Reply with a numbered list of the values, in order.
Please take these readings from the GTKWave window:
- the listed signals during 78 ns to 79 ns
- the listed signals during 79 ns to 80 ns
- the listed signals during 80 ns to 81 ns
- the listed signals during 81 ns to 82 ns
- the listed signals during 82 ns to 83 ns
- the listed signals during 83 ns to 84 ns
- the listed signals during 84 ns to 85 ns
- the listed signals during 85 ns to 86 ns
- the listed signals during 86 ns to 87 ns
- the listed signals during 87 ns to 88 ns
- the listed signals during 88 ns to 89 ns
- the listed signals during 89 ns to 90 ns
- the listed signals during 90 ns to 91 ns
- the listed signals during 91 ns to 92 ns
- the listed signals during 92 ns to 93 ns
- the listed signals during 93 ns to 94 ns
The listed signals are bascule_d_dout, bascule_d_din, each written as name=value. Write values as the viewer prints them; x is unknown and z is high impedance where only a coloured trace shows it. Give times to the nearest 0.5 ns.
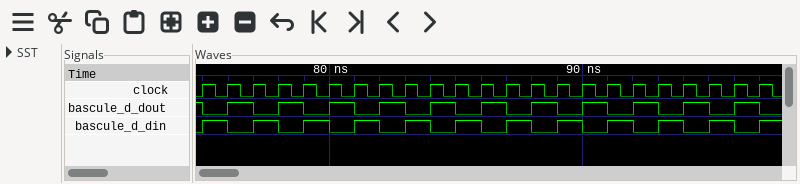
1. bascule_d_dout=1, bascule_d_din=0
2. bascule_d_dout=0, bascule_d_din=1
3. bascule_d_dout=1, bascule_d_din=0
4. bascule_d_dout=0, bascule_d_din=1
5. bascule_d_dout=1, bascule_d_din=0
6. bascule_d_dout=0, bascule_d_din=1
7. bascule_d_dout=1, bascule_d_din=0
8. bascule_d_dout=0, bascule_d_din=1
9. bascule_d_dout=1, bascule_d_din=0
10. bascule_d_dout=0, bascule_d_din=1
11. bascule_d_dout=1, bascule_d_din=0
12. bascule_d_dout=0, bascule_d_din=1
13. bascule_d_dout=1, bascule_d_din=0
14. bascule_d_dout=0, bascule_d_din=1
15. bascule_d_dout=1, bascule_d_din=0
16. bascule_d_dout=0, bascule_d_din=1
